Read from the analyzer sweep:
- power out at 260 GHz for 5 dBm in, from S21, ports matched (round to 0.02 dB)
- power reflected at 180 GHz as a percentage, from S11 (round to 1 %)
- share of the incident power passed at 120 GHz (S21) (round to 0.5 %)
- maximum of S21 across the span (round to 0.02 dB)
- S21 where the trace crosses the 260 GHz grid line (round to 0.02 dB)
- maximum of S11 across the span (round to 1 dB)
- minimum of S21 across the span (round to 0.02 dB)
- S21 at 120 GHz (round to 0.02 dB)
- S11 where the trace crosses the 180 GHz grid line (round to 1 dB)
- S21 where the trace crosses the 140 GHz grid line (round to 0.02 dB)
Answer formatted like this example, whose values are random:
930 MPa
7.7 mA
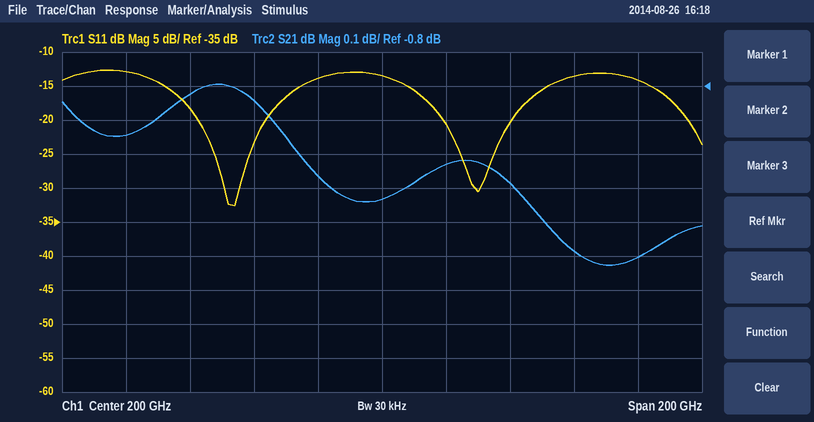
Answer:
3.72 dBm
4 %
80.5 %
-0.80 dB
-1.28 dB
-13 dB
-1.32 dB
-0.94 dB
-14 dB
-0.82 dB
